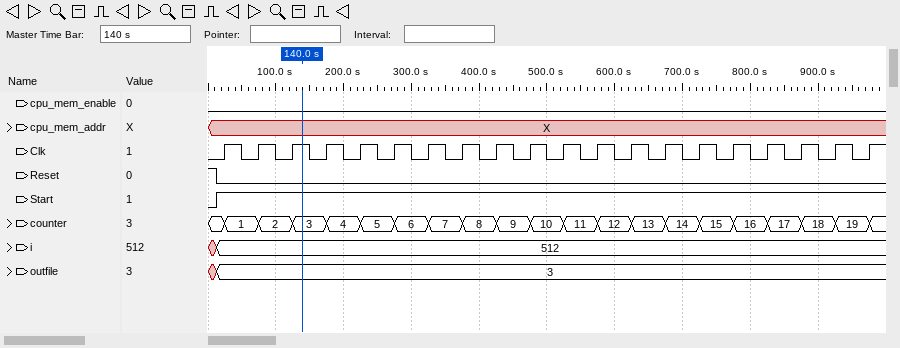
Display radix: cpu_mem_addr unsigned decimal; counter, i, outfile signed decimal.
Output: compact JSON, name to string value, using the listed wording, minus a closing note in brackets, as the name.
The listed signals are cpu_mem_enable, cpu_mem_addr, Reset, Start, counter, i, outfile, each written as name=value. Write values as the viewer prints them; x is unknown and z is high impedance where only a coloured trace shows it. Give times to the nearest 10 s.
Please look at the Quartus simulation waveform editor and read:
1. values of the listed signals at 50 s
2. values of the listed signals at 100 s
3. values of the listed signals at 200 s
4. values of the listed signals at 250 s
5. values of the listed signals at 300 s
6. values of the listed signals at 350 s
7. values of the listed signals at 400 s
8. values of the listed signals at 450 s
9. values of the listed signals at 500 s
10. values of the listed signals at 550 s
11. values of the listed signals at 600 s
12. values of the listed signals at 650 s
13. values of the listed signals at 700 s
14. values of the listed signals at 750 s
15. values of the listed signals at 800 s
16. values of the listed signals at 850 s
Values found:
{"values of the listed signals at 50 s": "cpu_mem_enable=0, cpu_mem_addr=X, Reset=0, Start=1, counter=1, i=512, outfile=3", "values of the listed signals at 100 s": "cpu_mem_enable=0, cpu_mem_addr=X, Reset=0, Start=1, counter=2, i=512, outfile=3", "values of the listed signals at 200 s": "cpu_mem_enable=0, cpu_mem_addr=X, Reset=0, Start=1, counter=4, i=512, outfile=3", "values of the listed signals at 250 s": "cpu_mem_enable=0, cpu_mem_addr=X, Reset=0, Start=1, counter=5, i=512, outfile=3", "values of the listed signals at 300 s": "cpu_mem_enable=0, cpu_mem_addr=X, Reset=0, Start=1, counter=6, i=512, outfile=3", "values of the listed signals at 350 s": "cpu_mem_enable=0, cpu_mem_addr=X, Reset=0, Start=1, counter=7, i=512, outfile=3", "values of the listed signals at 400 s": "cpu_mem_enable=0, cpu_mem_addr=X, Reset=0, Start=1, counter=8, i=512, outfile=3", "values of the listed signals at 450 s": "cpu_mem_enable=0, cpu_mem_addr=X, Reset=0, Start=1, counter=9, i=512, outfile=3", "values of the listed signals at 500 s": "cpu_mem_enable=0, cpu_mem_addr=X, Reset=0, Start=1, counter=10, i=512, outfile=3", "values of the listed signals at 550 s": "cpu_mem_enable=0, cpu_mem_addr=X, Reset=0, Start=1, counter=11, i=512, outfile=3", "values of the listed signals at 600 s": "cpu_mem_enable=0, cpu_mem_addr=X, Reset=0, Start=1, counter=12, i=512, outfile=3", "values of the listed signals at 650 s": "cpu_mem_enable=0, cpu_mem_addr=X, Reset=0, Start=1, counter=13, i=512, outfile=3", "values of the listed signals at 700 s": "cpu_mem_enable=0, cpu_mem_addr=X, Reset=0, Start=1, counter=14, i=512, outfile=3", "values of the listed signals at 750 s": "cpu_mem_enable=0, cpu_mem_addr=X, Reset=0, Start=1, counter=15, i=512, outfile=3", "values of the listed signals at 800 s": "cpu_mem_enable=0, cpu_mem_addr=X, Reset=0, Start=1, counter=16, i=512, outfile=3", "values of the listed signals at 850 s": "cpu_mem_enable=0, cpu_mem_addr=X, Reset=0, Start=1, counter=17, i=512, outfile=3"}
